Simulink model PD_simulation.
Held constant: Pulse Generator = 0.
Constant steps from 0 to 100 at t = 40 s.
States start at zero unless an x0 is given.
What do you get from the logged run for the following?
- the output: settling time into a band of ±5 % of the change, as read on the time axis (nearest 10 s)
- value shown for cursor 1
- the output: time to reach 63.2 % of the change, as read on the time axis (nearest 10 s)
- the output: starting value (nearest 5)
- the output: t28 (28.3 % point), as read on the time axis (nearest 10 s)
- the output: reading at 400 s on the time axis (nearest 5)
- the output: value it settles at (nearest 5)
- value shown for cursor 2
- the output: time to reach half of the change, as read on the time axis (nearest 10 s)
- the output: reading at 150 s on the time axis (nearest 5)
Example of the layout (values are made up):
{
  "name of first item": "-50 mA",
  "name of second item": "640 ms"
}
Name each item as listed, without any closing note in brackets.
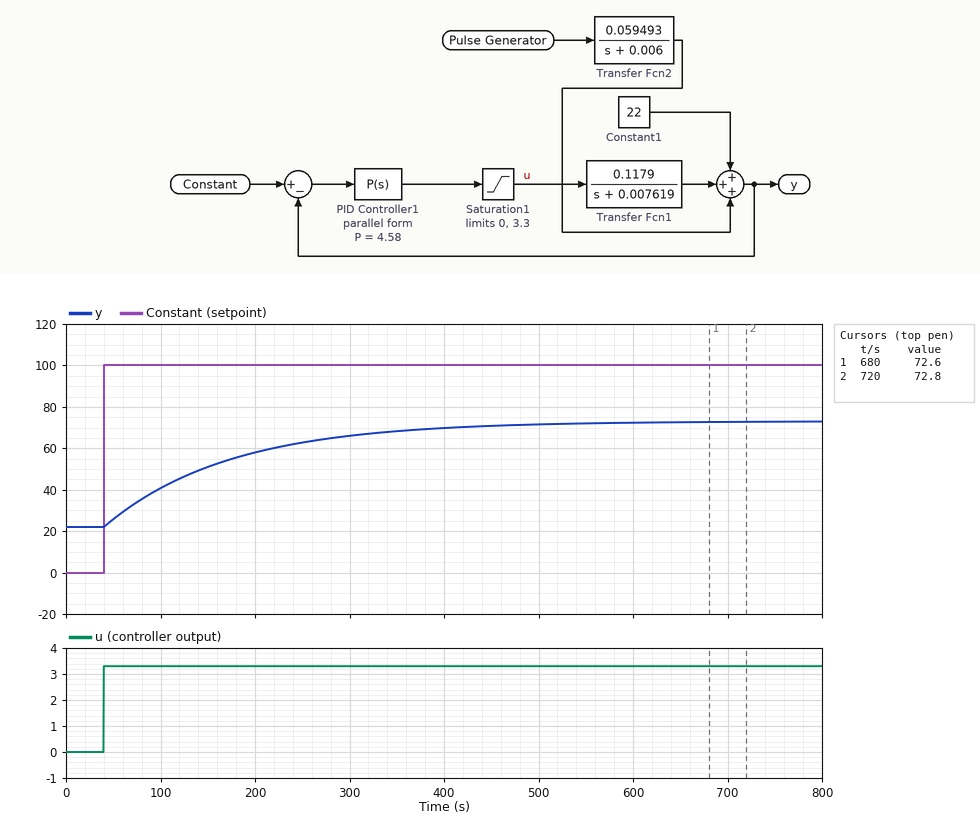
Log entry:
{
  "the output: settling time into a band of ±5 % of the change, as read on the time axis": "430 s",
  "value shown for cursor 1": "72.6",
  "the output: time to reach 63.2 % of the change, as read on the time axis": "170 s",
  "the output: starting value": "20",
  "the output: t28 (28.3 % point), as read on the time axis": "80 s",
  "the output: reading at 400 s on the time axis": "70",
  "the output: value it settles at": "75",
  "value shown for cursor 2": "72.8",
  "the output: time to reach half of the change, as read on the time axis": "130 s",
  "the output: reading at 150 s on the time axis": "50"
}
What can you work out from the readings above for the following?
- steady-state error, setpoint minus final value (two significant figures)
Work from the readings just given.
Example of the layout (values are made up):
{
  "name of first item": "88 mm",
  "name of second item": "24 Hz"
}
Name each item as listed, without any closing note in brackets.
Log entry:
{
  "steady-state error, setpoint minus final value": "25"
}
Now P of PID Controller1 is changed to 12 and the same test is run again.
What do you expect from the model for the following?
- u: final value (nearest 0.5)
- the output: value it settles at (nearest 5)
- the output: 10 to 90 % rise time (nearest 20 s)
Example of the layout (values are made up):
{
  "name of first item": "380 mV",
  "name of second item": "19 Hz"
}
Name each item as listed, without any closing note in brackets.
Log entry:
{
  "u: final value": "3.5",
  "the output: value it settles at": "75",
  "the output: 10 to 90 % rise time": "280 s"
}
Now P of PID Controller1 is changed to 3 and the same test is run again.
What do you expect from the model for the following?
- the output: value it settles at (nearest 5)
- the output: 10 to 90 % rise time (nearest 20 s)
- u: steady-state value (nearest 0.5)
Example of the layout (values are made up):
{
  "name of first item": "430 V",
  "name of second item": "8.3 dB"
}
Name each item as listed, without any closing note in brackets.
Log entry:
{
  "the output: value it settles at": "75",
  "the output: 10 to 90 % rise time": "280 s",
  "u: steady-state value": "3.5"
}
